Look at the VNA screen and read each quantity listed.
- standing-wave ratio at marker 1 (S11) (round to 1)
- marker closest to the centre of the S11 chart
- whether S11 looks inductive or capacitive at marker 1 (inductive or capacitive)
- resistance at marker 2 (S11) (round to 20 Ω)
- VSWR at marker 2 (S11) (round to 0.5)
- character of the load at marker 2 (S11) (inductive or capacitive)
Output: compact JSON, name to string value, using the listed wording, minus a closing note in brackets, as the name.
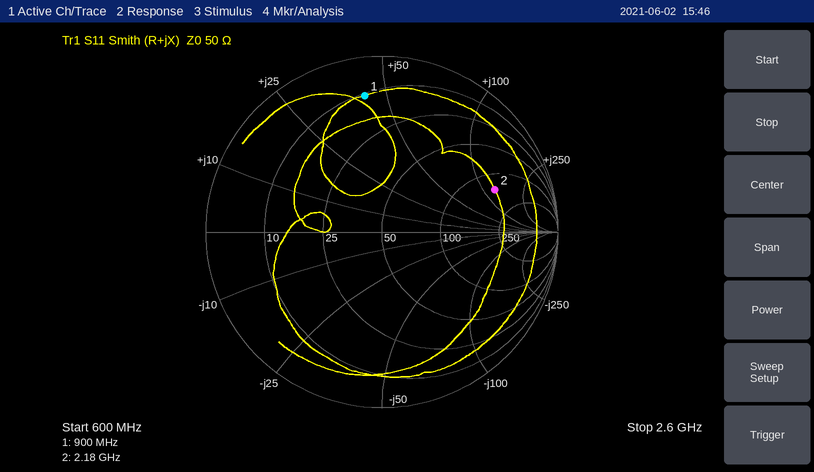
{"standing-wave ratio at marker 1 (S11)": "8", "marker closest to the centre of the S11 chart": "marker 2", "whether S11 looks inductive or capacitive at marker 1": "inductive", "resistance at marker 2 (S11)": "140 Ω", "VSWR at marker 2 (S11)": "5.5", "character of the load at marker 2 (S11)": "inductive"}
